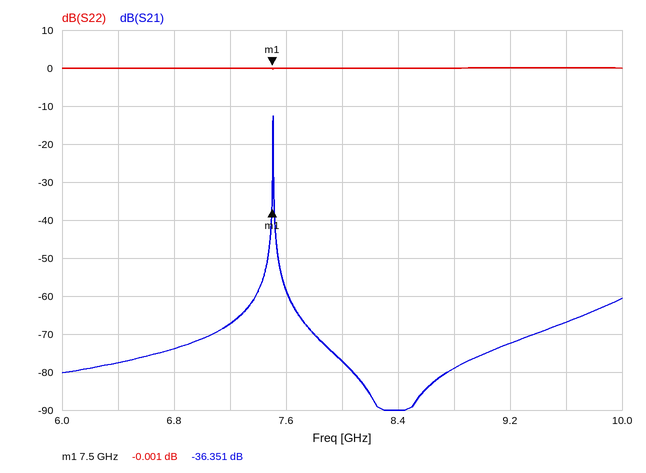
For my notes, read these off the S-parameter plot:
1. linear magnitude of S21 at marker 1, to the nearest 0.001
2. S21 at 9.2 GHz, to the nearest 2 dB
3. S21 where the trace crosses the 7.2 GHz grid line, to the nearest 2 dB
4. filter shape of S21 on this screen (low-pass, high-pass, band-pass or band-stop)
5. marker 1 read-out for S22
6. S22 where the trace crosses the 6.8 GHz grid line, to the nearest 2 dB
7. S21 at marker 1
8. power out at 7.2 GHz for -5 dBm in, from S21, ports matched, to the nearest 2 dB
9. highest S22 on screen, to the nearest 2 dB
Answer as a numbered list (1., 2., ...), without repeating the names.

1. 0.015
2. -72 dB
3. -68 dB
4. band-pass
5. -0.001 dB
6. 0 dB
7. -36.351 dB
8. -72 dBm
9. 0 dB
